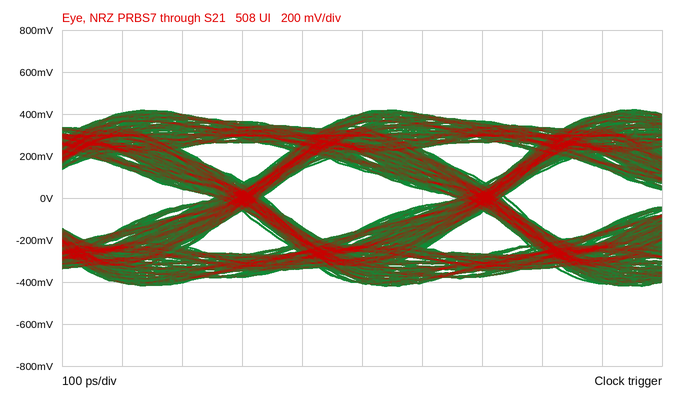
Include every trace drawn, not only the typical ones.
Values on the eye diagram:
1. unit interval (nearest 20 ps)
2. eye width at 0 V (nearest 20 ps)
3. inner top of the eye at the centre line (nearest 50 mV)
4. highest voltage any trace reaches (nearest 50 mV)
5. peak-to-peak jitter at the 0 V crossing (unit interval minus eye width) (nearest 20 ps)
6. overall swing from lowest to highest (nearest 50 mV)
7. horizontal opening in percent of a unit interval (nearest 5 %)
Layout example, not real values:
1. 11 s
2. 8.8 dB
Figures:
1. 400 ps
2. 320 ps
3. 150 mV
4. 400 mV
5. 80 ps
6. 850 mV
7. 80 %
